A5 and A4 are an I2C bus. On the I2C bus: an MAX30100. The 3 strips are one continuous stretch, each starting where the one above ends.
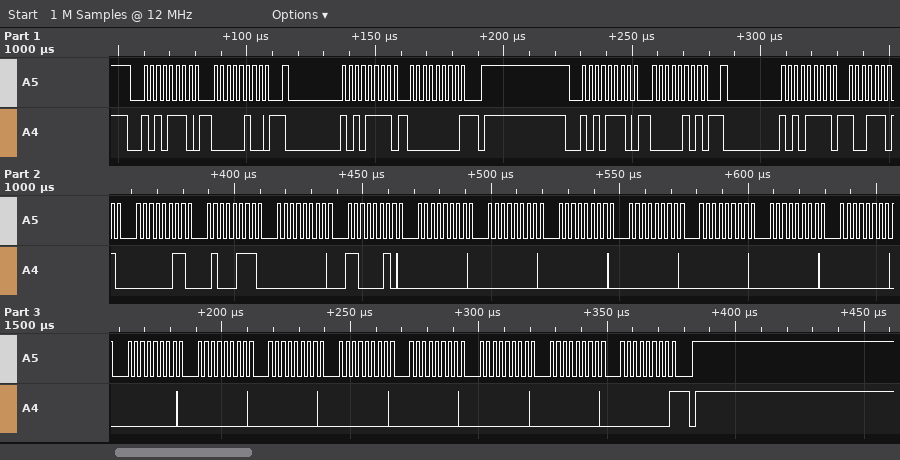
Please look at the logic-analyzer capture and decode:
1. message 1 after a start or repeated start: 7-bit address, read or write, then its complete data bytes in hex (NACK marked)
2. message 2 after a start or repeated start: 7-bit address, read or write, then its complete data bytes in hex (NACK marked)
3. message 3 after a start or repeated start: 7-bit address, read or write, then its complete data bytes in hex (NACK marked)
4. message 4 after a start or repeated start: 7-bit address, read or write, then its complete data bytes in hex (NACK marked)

0x57 write: 04
0x57 read: 00 NACK
0x57 write: 05
0x57 read: 9D 03 47 00 C2 00 00 00 00 00 00 00 00 00 00 00 00 00 00 00 NACK
